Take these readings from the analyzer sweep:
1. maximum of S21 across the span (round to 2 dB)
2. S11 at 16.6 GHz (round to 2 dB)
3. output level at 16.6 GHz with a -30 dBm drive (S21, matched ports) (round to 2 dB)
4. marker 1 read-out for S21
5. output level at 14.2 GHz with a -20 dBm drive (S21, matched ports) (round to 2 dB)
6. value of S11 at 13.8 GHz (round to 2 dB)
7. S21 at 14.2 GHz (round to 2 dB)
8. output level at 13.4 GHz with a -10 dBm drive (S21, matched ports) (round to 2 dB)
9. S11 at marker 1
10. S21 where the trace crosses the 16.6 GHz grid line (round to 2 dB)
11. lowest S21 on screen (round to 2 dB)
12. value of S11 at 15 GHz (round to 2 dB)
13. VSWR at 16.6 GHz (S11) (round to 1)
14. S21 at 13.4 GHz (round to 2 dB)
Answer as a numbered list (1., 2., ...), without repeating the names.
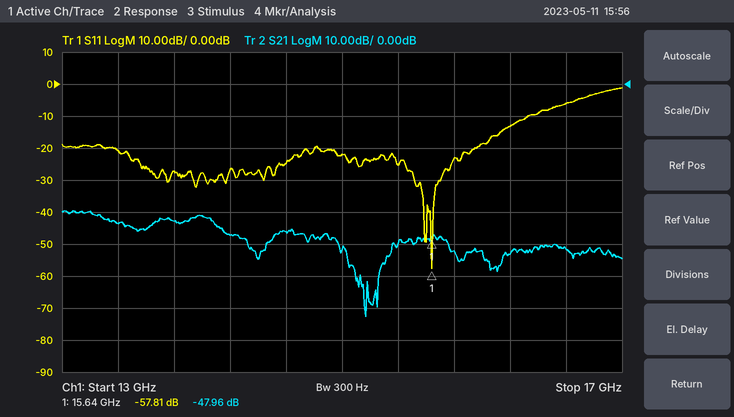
1. -40 dB
2. -6 dB
3. -82 dBm
4. -47.96 dB
5. -68 dBm
6. -28 dB
7. -48 dB
8. -54 dBm
9. -57.81 dB
10. -52 dB
11. -72 dB
12. -22 dB
13. 3
14. -44 dB
